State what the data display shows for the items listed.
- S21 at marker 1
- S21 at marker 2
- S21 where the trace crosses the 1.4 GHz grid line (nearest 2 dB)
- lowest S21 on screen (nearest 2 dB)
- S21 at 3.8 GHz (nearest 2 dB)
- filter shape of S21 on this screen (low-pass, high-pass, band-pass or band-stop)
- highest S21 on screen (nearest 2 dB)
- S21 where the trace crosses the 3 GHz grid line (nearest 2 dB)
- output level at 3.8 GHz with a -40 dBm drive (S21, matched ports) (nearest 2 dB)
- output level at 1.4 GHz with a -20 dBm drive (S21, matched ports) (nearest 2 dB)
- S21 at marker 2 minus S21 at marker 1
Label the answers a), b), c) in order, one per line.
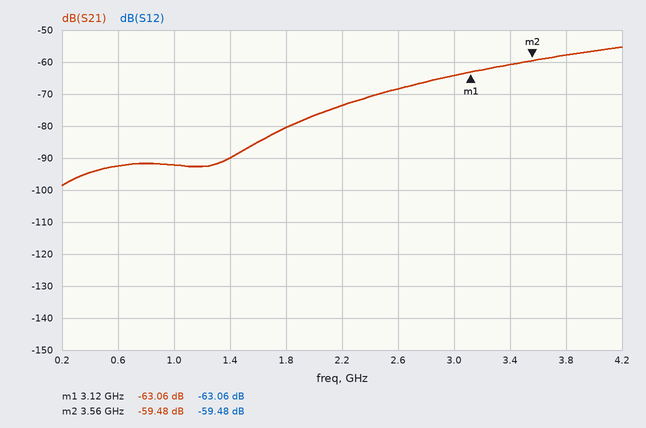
a) -63.06 dB
b) -59.48 dB
c) -90 dB
d) -98 dB
e) -58 dB
f) high-pass
g) -56 dB
h) -64 dB
i) -98 dBm
j) -110 dBm
k) 3.58 dB
